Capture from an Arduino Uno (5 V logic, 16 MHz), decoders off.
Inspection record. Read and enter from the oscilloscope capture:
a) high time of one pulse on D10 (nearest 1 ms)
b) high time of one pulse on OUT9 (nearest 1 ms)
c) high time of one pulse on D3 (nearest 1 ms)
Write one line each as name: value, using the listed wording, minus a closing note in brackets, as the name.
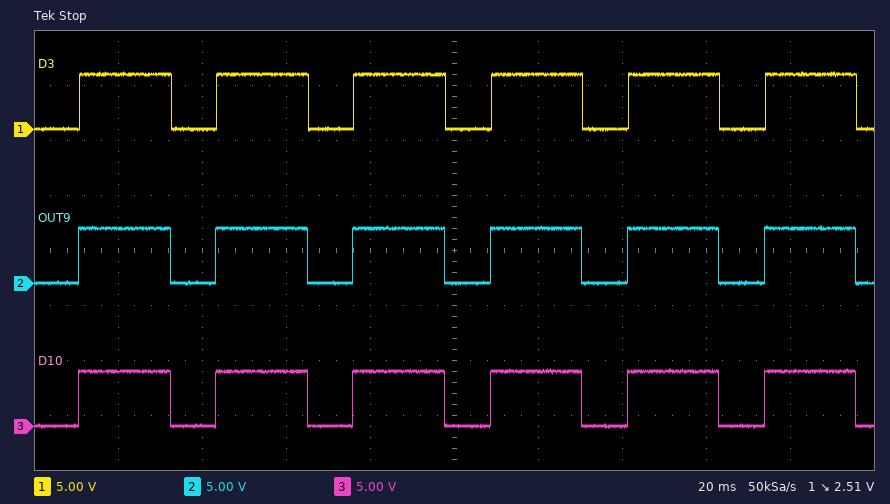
high time of one pulse on D10: 22 ms
high time of one pulse on OUT9: 22 ms
high time of one pulse on D3: 22 ms
